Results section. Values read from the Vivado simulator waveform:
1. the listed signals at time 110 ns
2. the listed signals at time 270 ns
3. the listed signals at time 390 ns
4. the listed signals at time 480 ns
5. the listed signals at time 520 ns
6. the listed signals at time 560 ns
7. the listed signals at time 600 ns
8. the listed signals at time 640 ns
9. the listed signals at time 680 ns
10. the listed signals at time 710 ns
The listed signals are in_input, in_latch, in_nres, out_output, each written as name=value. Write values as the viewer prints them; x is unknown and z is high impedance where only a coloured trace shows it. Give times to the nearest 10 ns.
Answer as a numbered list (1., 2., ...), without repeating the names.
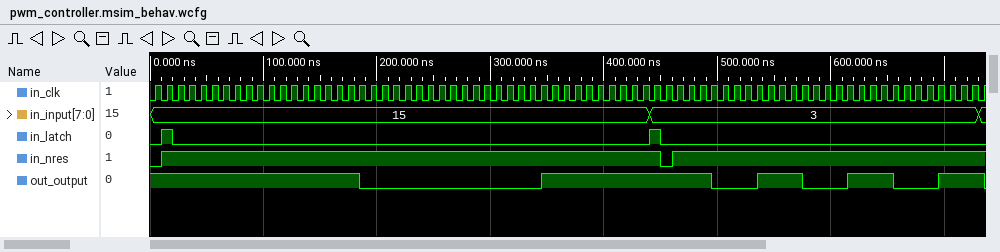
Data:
1. in_input=15, in_latch=0, in_nres=1, out_output=1
2. in_input=15, in_latch=0, in_nres=1, out_output=0
3. in_input=15, in_latch=0, in_nres=1, out_output=1
4. in_input=3, in_latch=0, in_nres=1, out_output=1
5. in_input=3, in_latch=0, in_nres=1, out_output=0
6. in_input=3, in_latch=0, in_nres=1, out_output=1
7. in_input=3, in_latch=0, in_nres=1, out_output=0
8. in_input=3, in_latch=0, in_nres=1, out_output=1
9. in_input=3, in_latch=0, in_nres=1, out_output=0
10. in_input=3, in_latch=0, in_nres=1, out_output=1
